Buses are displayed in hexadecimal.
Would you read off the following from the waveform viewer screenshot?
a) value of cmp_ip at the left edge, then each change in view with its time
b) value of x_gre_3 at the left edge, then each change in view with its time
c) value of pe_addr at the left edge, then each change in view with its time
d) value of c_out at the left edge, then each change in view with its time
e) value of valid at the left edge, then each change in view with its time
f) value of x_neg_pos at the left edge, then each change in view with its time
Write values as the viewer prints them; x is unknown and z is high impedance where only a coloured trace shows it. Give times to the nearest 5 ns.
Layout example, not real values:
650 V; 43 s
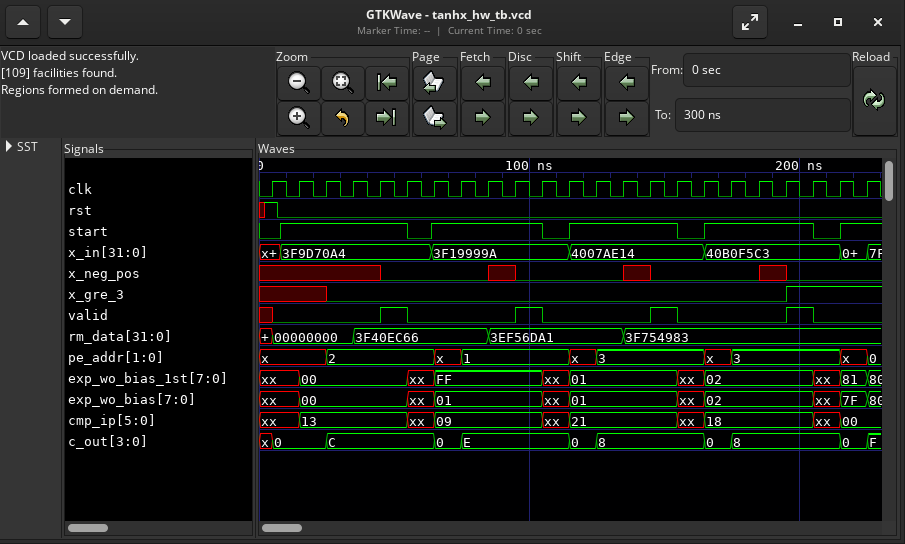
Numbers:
xx, 13 at 15 ns, xx at 55 ns, 09 at 65 ns, xx at 105 ns, 21 at 115 ns, xx at 155 ns, 18 at 165 ns, xx at 205 ns, 00 at 215 ns; x, 0 at 25 ns, 1 at 195 ns; x, 2 at 25 ns, x at 65 ns, 1 at 75 ns, x at 115 ns, 3 at 125 ns, x at 165 ns, 3 at 175 ns, x at 215 ns, 0 at 225 ns; x, 0 at 5 ns, C at 25 ns, 0 at 65 ns, E at 75 ns, 0 at 115 ns, 8 at 125 ns, 0 at 165 ns, 8 at 175 ns, 0 at 215 ns, F at 225 ns; x, 0 at 5 ns, 1 at 45 ns, 0 at 55 ns, 1 at 95 ns, 0 at 105 ns, 1 at 145 ns, 0 at 155 ns, 1 at 195 ns, 0 at 205 ns; x, 0 at 45 ns, x at 85 ns, 0 at 95 ns, x at 135 ns, 0 at 145 ns, x at 185 ns, 0 at 195 ns
